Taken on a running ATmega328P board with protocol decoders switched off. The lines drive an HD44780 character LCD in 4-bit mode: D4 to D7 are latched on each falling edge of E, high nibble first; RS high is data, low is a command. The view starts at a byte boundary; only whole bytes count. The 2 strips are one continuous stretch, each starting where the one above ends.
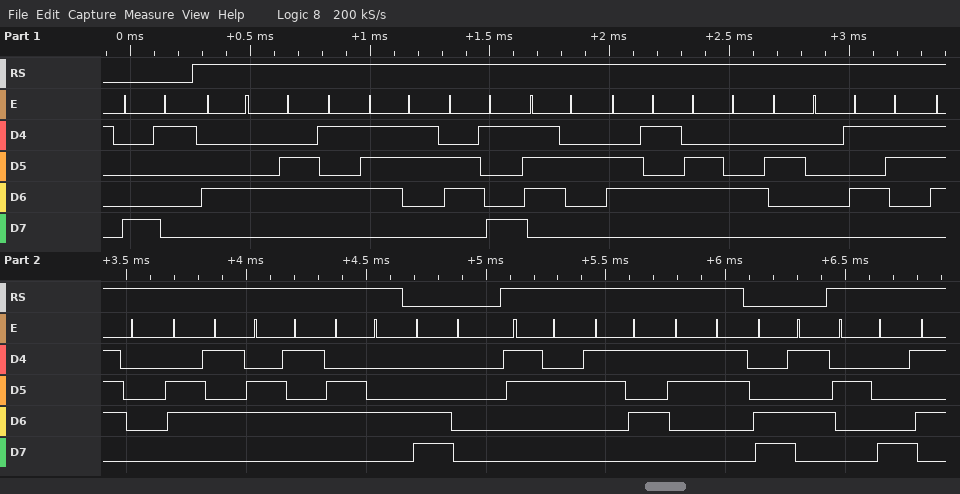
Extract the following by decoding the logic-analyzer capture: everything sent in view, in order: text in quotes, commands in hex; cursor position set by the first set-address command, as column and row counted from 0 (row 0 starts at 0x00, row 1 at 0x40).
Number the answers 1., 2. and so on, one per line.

1. 0x81 "Desired Speed" 0xC0 "253" 0xC5 "("
2. column 1, row 0
